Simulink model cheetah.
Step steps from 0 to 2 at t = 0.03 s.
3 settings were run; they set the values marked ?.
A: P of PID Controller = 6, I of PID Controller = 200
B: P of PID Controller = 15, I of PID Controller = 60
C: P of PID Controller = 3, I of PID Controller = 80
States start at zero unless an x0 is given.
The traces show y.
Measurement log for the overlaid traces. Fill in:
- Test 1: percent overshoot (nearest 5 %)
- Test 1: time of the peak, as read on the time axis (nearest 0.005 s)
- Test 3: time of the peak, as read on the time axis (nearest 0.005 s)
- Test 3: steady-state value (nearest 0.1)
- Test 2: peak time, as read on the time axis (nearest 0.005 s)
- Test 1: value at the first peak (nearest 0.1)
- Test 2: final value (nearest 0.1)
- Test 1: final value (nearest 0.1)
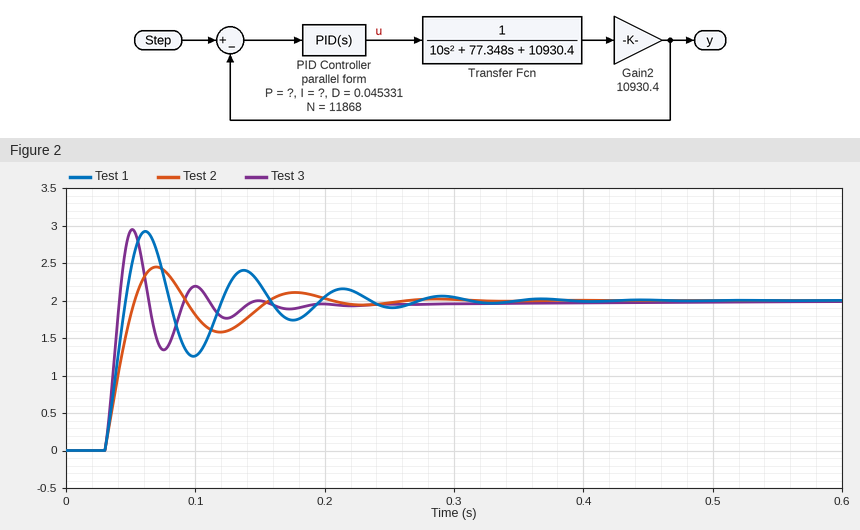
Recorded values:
45 %
0.060 s
0.050 s
2.0
0.070 s
2.9
2.0
2.0
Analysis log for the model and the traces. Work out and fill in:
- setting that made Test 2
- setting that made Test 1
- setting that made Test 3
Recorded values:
C
A
B
